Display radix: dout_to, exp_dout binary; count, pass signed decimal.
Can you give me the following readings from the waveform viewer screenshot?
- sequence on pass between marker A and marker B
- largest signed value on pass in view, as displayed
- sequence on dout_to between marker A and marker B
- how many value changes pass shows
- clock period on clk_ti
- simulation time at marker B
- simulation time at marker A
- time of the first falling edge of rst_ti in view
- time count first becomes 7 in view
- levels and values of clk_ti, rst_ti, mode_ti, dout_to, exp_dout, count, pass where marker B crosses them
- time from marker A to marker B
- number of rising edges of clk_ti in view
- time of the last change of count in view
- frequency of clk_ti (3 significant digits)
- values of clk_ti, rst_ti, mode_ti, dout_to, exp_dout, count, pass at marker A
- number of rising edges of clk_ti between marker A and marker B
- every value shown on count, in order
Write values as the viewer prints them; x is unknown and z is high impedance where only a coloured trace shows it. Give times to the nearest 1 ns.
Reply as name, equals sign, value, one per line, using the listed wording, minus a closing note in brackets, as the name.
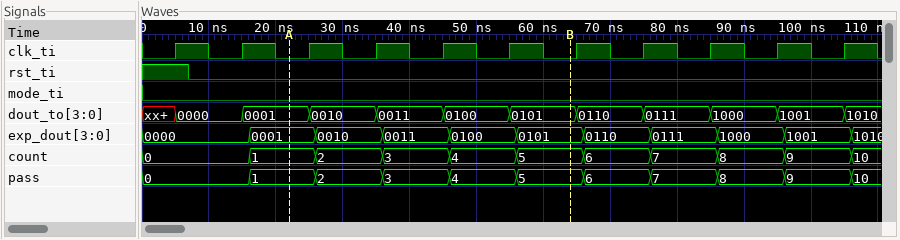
sequence on pass between marker A and marker B = 1, 2, 3, 4, 5
largest signed value on pass in view, as displayed = 10
sequence on dout_to between marker A and marker B = 0001, 0010, 0011, 0100, 0101
how many value changes pass shows = 10
clock period on clk_ti = 10 ns
simulation time at marker B = 64 ns
simulation time at marker A = 22 ns
time of the first falling edge of rst_ti in view = 7 ns
time count first becomes 7 in view = 76 ns
levels and values of clk_ti, rst_ti, mode_ti, dout_to, exp_dout, count, pass where marker B crosses them = clk_ti=0, rst_ti=0, mode_ti=0, dout_to=0101, exp_dout=0101, count=5, pass=5
time from marker A to marker B = 42 ns
number of rising edges of clk_ti in view = 11
time of the last change of count in view = 106 ns
frequency of clk_ti = 100 MHz
values of clk_ti, rst_ti, mode_ti, dout_to, exp_dout, count, pass at marker A = clk_ti=0, rst_ti=0, mode_ti=0, dout_to=0001, exp_dout=0001, count=1, pass=1
number of rising edges of clk_ti between marker A and marker B = 4
every value shown on count, in order = 0, 1, 2, 3, 4, 5, 6, 7, 8, 9, 10
